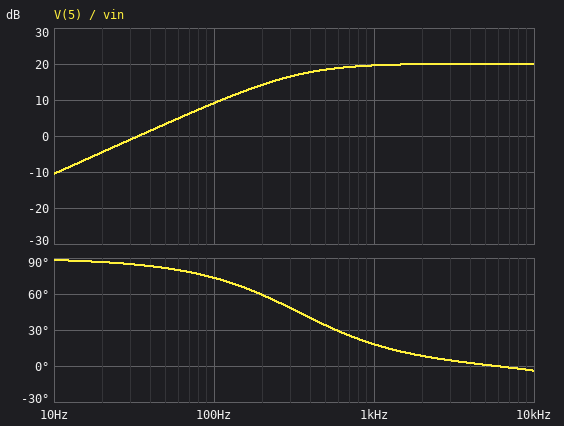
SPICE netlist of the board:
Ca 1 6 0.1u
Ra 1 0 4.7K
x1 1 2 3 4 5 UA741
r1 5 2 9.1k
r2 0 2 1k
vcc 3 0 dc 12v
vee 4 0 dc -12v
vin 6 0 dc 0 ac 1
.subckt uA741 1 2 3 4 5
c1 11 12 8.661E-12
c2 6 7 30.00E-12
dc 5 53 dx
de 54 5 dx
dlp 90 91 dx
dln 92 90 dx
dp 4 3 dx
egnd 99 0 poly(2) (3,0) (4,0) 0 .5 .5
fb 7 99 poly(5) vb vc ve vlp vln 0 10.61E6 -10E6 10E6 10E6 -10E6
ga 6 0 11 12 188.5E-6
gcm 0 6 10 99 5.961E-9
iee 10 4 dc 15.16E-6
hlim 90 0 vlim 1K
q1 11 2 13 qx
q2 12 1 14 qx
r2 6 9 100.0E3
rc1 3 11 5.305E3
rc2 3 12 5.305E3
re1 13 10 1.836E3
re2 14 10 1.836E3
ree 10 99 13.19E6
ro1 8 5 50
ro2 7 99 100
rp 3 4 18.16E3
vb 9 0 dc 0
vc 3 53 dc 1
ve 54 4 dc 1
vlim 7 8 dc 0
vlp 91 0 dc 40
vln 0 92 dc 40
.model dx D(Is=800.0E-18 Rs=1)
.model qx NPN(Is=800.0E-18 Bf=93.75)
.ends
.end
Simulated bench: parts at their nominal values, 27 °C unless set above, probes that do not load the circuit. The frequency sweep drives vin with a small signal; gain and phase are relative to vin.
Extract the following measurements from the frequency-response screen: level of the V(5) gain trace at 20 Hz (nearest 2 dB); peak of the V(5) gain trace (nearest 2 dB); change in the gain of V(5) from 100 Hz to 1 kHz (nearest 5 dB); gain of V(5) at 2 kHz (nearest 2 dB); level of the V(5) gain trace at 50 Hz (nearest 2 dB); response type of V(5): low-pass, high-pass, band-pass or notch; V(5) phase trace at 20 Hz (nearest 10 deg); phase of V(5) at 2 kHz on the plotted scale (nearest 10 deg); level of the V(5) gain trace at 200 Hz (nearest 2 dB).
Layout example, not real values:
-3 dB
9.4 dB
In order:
-4 dB
20 dB
10 dB
20 dB
4 dB
high-pass
90 deg
10 deg
14 dB
